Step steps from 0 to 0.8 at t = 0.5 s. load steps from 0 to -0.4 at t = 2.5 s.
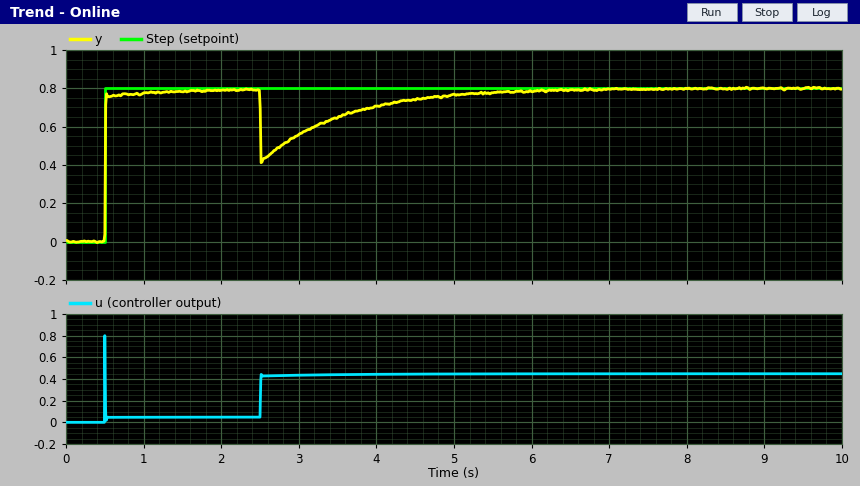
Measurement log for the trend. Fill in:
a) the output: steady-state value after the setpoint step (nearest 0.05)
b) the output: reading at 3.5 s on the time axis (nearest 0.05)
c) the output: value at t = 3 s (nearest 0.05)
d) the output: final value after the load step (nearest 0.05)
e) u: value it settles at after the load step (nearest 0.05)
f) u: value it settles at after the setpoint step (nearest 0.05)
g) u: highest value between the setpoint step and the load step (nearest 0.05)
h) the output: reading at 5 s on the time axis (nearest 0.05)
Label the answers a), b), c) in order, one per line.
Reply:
a) 0.80
b) 0.65
c) 0.55
d) 0.80
e) 0.45
f) 0.05
g) 0.80
h) 0.75
